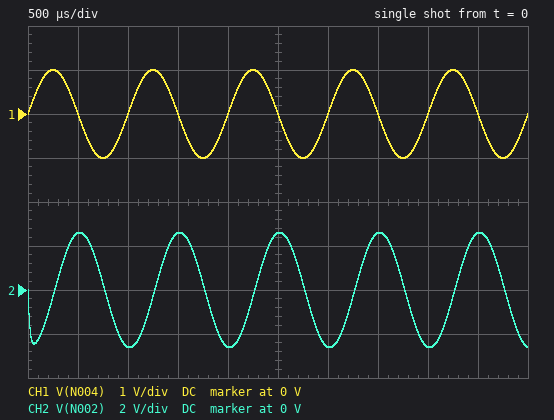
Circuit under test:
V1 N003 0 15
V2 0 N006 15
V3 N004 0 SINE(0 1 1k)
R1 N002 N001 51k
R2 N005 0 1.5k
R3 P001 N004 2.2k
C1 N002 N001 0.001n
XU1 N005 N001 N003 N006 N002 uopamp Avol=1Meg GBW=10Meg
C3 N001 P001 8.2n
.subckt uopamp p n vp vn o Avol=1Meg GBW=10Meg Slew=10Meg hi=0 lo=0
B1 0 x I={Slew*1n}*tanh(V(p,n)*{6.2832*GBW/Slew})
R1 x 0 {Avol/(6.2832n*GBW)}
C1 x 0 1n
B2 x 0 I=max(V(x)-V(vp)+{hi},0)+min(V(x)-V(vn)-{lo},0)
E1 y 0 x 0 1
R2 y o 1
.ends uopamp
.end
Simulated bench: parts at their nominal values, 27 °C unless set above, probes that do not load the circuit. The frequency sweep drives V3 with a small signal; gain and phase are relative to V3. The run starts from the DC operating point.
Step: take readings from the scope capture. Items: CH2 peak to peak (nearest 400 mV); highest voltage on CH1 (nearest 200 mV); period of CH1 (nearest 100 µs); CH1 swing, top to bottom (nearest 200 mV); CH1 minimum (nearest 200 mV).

5.2 V
1.0 V
1.0 ms
2.0 V
-1.0 V
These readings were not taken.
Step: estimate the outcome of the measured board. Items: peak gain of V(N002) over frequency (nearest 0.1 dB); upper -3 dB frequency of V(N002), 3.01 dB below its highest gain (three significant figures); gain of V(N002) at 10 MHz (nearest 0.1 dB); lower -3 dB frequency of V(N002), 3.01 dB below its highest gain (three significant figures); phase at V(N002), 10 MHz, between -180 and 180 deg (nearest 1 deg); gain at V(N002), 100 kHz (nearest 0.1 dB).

27.3 dB
377 kHz
-1.5 dB
8.59 kHz
85 deg
27.1 dB
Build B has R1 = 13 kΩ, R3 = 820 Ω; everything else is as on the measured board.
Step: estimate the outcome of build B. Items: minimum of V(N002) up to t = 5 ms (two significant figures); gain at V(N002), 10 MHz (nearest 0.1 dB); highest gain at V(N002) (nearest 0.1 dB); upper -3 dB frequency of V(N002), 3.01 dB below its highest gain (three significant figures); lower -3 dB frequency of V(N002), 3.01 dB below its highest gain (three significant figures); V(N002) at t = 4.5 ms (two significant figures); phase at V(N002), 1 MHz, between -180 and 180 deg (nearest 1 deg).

-670 mV
-0.9 dB
24.0 dB
592 kHz
22.7 kHz
670 mV
120 deg
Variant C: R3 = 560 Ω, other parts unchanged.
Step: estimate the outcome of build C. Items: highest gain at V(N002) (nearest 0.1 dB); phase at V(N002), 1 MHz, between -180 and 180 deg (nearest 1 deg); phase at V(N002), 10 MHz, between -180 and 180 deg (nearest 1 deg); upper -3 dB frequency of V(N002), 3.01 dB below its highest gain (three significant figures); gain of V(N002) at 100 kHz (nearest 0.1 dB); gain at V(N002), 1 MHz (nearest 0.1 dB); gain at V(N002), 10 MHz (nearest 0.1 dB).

39.1 dB
96 deg
89 deg
134 kHz
37.7 dB
19.6 dB
-0.4 dB
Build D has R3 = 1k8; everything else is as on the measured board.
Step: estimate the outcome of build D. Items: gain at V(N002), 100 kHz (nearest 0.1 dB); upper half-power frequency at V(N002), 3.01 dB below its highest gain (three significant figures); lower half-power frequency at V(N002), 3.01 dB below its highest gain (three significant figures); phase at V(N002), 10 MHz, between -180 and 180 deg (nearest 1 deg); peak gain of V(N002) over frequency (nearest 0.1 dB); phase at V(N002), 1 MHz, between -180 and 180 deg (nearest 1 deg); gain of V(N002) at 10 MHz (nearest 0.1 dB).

28.8 dB
320 kHz
10.4 kHz
86 deg
29.0 dB
107 deg
-1.2 dB
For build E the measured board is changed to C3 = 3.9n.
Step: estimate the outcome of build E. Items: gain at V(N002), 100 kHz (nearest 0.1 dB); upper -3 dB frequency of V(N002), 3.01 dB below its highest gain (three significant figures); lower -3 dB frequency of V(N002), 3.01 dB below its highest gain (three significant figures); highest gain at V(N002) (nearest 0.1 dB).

27.2 dB
387 kHz
17.6 kHz
27.2 dB
